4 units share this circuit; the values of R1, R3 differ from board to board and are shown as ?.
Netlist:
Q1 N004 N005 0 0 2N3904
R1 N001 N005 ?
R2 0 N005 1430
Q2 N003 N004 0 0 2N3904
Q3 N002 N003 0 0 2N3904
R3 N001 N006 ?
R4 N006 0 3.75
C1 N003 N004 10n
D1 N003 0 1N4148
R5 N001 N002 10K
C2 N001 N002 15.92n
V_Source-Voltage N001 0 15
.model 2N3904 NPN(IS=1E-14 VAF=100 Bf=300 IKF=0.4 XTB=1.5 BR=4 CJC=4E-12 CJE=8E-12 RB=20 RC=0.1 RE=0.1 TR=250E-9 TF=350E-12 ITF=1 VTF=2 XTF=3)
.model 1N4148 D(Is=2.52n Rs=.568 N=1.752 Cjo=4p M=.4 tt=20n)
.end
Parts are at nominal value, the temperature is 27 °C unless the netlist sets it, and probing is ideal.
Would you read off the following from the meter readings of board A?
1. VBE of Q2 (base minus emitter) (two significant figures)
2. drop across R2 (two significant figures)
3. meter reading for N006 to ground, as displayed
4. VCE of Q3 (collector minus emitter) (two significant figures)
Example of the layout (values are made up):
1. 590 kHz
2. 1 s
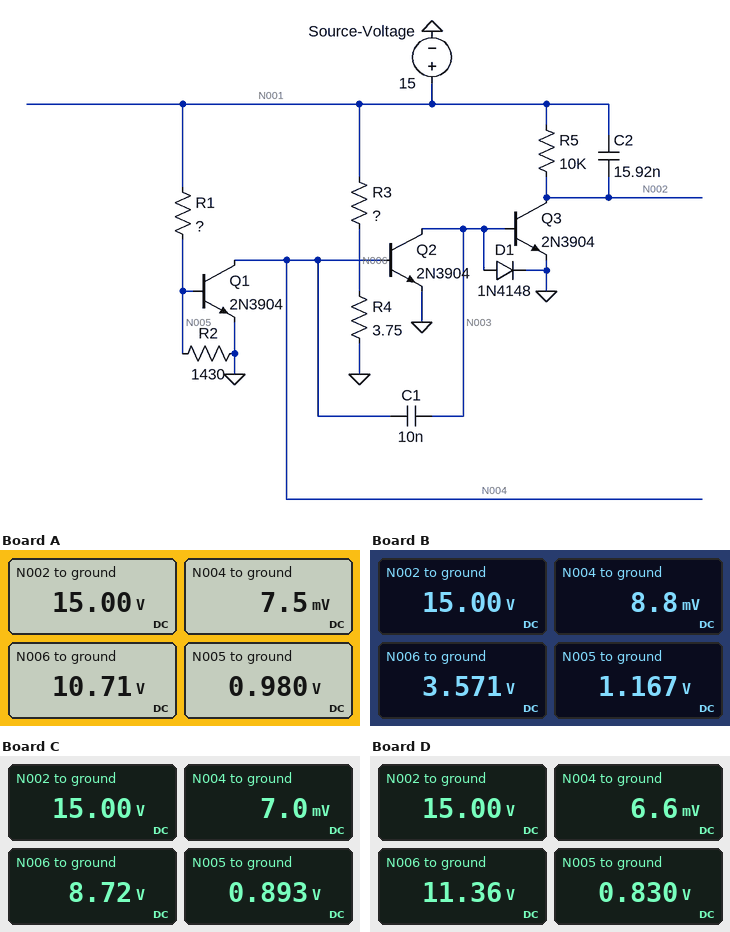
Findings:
1. 7.5 mV
2. 980 mV
3. 10.71 V
4. 15 V
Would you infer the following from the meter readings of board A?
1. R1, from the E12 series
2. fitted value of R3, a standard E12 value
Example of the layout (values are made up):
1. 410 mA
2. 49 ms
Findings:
1. 1.2 kΩ
2. 1.5 Ω
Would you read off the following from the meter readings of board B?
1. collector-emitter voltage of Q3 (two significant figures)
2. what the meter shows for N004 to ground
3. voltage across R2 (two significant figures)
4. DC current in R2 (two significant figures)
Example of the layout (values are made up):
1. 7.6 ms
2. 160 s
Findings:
1. 15 V
2. 8.8 mV
3. 1.2 V
4. 820 µA
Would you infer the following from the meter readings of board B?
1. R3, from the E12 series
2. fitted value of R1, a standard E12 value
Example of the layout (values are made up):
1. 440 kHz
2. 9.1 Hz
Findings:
1. 12 Ω
2. 680 Ω
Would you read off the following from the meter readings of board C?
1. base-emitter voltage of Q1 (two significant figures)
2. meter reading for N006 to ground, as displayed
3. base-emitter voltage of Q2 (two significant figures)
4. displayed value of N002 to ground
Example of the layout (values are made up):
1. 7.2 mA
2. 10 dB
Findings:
1. 890 mV
2. 8.72 V
3. 7.0 mV
4. 15.00 V
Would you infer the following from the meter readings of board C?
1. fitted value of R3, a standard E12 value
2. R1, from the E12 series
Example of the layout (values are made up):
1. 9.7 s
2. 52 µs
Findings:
1. 2.7 Ω
2. 1.8 kΩ
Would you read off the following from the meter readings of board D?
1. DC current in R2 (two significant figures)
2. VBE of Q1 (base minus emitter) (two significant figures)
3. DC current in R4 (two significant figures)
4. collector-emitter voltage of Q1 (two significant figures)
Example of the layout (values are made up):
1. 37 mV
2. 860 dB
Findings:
1. 580 µA
2. 830 mV
3. 3.0 A
4. 6.6 mV
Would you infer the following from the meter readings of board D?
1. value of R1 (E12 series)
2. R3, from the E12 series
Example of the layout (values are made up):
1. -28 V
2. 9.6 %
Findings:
1. 2.7 kΩ
2. 1.2 Ω
